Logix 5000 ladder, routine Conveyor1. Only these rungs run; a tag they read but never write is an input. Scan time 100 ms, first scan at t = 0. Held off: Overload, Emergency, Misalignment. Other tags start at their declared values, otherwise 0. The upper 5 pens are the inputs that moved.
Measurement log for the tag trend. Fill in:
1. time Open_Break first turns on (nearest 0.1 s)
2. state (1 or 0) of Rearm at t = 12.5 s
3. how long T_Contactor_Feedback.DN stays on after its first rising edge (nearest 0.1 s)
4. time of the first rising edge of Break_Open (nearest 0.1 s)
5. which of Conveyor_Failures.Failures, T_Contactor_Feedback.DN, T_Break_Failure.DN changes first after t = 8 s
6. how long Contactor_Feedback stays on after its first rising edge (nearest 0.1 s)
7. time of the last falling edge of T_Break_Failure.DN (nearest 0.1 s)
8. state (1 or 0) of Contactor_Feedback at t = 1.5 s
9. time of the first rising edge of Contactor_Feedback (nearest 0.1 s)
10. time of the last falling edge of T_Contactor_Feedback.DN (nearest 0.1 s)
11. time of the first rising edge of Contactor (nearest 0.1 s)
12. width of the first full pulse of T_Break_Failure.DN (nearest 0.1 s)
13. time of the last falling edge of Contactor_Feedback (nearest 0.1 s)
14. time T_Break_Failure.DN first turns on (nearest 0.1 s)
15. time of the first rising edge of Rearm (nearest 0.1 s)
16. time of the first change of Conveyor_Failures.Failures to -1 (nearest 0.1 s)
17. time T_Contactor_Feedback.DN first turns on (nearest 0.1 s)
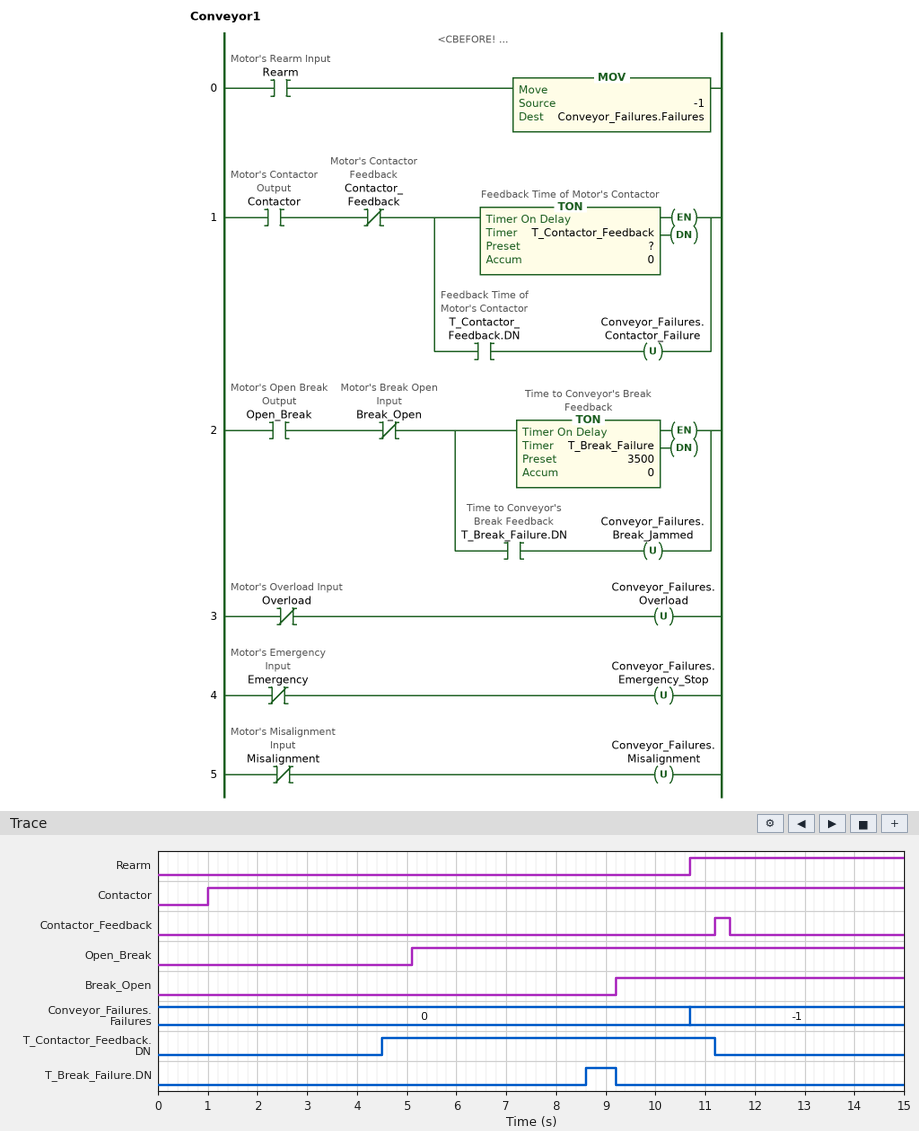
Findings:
5.1 s
1
6.7 s
9.2 s
T_Break_Failure.DN
0.3 s
9.2 s
0
11.2 s
11.2 s
1.0 s
0.6 s
11.5 s
8.6 s
10.7 s
10.7 s
4.5 s
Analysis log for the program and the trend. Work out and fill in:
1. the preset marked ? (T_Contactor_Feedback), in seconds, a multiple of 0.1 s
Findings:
3.5 s
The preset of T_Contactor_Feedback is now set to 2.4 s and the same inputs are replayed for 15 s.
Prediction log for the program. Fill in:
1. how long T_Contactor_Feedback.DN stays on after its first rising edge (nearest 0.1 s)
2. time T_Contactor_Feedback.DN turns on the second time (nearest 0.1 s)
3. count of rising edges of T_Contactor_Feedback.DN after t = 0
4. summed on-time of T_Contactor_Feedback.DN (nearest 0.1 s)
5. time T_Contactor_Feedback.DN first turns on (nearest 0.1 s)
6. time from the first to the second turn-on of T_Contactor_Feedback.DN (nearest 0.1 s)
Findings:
7.8 s
13.9 s
2
8.9 s
3.4 s
10.5 s
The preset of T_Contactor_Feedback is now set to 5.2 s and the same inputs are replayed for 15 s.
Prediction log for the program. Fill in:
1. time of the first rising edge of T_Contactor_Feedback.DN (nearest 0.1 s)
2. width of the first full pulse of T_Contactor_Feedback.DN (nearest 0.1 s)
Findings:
6.2 s
5.0 s
